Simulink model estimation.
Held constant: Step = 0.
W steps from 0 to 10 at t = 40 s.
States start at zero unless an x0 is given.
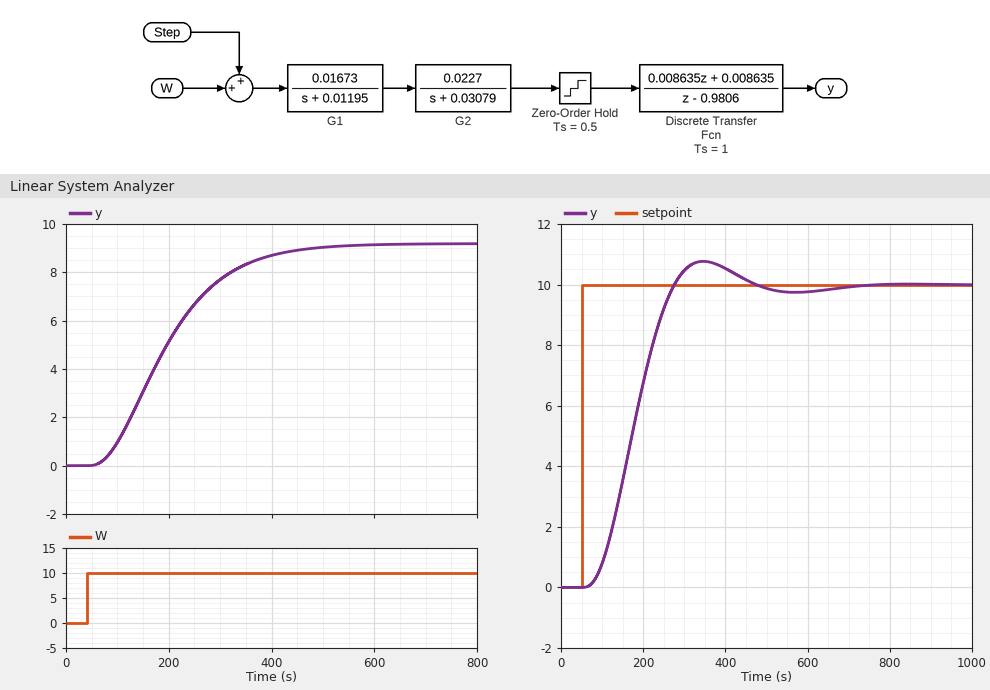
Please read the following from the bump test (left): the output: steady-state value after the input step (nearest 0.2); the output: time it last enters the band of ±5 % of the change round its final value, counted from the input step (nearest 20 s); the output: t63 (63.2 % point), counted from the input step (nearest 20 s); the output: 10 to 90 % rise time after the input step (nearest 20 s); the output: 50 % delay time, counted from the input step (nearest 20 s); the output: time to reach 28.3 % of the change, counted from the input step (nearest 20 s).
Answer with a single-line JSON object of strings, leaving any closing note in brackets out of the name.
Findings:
{"the output: steady-state value after the input step": "9.2", "the output: time it last enters the band of ±5 % of the change round its final value, counted from the input step": "360 s", "the output: t63 (63.2 % point), counted from the input step": "180 s", "the output: 10 to 90 % rise time after the input step": "240 s", "the output: 50 % delay time, counted from the input step": "140 s", "the output: time to reach 28.3 % of the change, counted from the input step": "100 s"}
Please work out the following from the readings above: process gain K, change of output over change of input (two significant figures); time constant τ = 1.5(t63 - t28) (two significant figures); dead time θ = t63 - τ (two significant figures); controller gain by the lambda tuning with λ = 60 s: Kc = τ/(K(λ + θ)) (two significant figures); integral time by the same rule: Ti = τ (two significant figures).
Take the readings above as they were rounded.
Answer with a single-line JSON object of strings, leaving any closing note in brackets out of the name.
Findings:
{"process gain K, change of output over change of input": "0.92", "time constant τ = 1.5(t63 - t28)": "120 s", "dead time θ = t63 - τ": "60 s", "controller gain by the lambda tuning with λ = 60 s: Kc = τ/(K(λ + θ))": "1.1", "integral time by the same rule: Ti = τ": "120 s"}
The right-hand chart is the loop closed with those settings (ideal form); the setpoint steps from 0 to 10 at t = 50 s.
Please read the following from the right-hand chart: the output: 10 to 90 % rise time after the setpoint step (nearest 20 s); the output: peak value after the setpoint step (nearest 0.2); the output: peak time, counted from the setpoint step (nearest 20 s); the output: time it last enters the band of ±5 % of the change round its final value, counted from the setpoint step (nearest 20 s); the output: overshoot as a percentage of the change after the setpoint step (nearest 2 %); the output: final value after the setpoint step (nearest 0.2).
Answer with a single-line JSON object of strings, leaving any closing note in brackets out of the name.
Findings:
{"the output: 10 to 90 % rise time after the setpoint step": "140 s", "the output: peak value after the setpoint step": "10.8", "the output: peak time, counted from the setpoint step": "300 s", "the output: time it last enters the band of ±5 % of the change round its final value, counted from the setpoint step": "360 s", "the output: overshoot as a percentage of the change after the setpoint step": "8 %", "the output: final value after the setpoint step": "10.0"}
